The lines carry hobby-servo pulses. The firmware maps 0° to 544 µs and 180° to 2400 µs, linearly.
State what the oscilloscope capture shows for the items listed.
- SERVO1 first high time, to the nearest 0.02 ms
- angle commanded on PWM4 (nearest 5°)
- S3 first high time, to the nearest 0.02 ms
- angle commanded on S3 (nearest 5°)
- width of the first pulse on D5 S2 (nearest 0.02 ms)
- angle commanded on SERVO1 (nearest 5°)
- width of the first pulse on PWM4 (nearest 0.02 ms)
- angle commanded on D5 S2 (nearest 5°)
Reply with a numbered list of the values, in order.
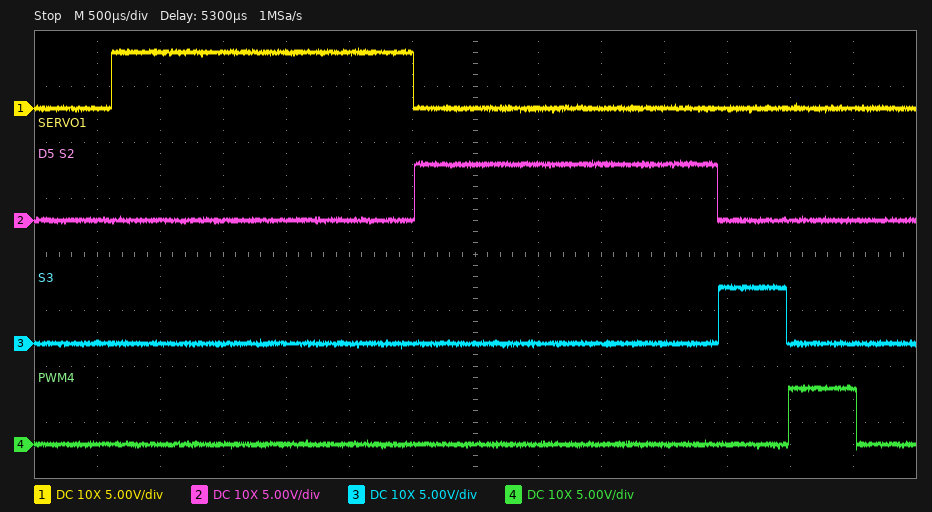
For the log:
1. 2.40 ms
2. 0°
3. 0.54 ms
4. 0°
5. 2.40 ms
6. 180°
7. 0.54 ms
8. 180°
